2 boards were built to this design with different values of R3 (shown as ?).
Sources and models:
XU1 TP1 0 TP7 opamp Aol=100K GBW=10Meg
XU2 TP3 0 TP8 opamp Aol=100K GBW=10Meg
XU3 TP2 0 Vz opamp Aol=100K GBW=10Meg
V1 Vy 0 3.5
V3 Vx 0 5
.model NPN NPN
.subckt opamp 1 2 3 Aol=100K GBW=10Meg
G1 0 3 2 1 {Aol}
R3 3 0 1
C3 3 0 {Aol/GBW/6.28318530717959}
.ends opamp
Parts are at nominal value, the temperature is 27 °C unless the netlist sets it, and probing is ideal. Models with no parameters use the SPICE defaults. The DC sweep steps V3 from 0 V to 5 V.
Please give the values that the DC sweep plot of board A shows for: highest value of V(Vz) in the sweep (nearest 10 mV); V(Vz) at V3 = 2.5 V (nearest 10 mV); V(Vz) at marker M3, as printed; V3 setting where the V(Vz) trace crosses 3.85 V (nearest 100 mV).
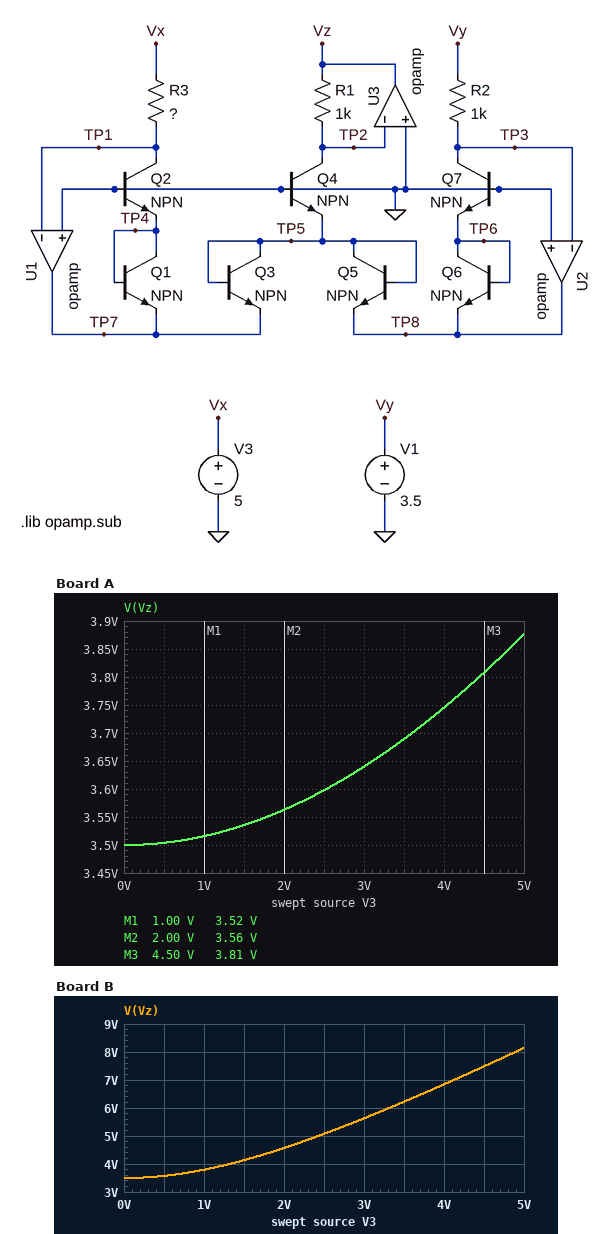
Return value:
3.88 V
3.60 V
3.81 V
4.8 V
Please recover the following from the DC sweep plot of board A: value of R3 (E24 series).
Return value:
3 kΩ
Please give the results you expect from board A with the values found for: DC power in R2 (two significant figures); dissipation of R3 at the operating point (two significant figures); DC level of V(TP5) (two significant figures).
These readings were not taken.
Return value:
12 mW
8.3 mW
-810 mV
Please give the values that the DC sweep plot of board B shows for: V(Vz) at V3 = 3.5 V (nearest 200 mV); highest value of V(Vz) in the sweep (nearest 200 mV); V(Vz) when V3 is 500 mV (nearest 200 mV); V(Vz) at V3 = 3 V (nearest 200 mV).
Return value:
6.2 V
8.2 V
3.6 V
5.6 V
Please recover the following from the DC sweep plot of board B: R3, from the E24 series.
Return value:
680 Ω
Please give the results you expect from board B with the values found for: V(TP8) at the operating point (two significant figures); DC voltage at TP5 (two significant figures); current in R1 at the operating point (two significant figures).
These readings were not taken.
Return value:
-1.6 V
-830 mV
8.1 mA
